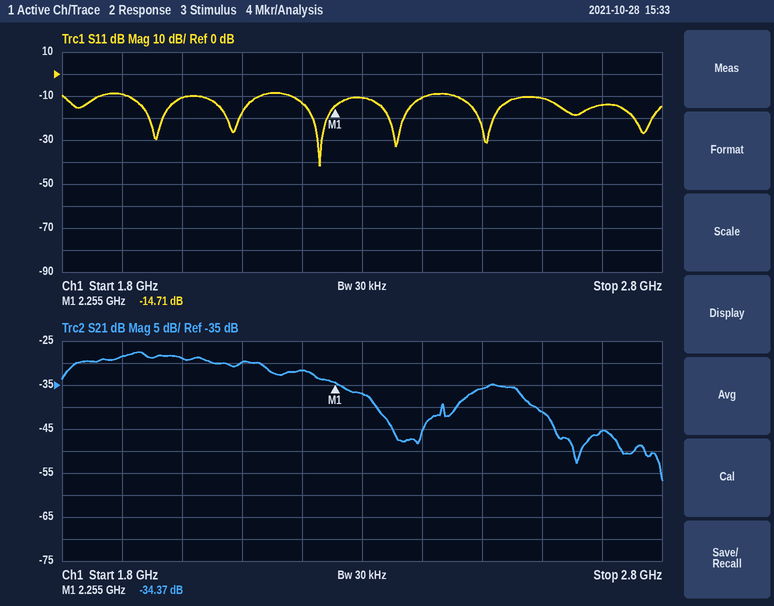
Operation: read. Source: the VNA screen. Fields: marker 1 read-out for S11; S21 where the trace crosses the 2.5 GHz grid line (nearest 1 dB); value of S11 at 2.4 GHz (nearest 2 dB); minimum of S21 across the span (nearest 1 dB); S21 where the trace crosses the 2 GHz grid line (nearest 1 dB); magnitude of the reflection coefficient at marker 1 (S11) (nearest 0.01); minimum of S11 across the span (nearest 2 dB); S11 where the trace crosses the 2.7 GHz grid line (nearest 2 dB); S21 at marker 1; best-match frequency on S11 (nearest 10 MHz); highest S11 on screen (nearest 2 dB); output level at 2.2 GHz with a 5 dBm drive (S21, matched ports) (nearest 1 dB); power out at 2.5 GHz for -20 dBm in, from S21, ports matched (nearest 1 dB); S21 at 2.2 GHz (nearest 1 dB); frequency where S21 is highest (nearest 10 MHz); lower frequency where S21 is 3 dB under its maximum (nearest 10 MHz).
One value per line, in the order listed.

-14.71 dB
-36 dB
-10 dB
-57 dB
-29 dB
0.18
-42 dB
-14 dB
-34.37 dB
2.23 GHz
-8 dB
-27 dBm
-56 dBm
-32 dB
1.93 GHz
1.82 GHz
